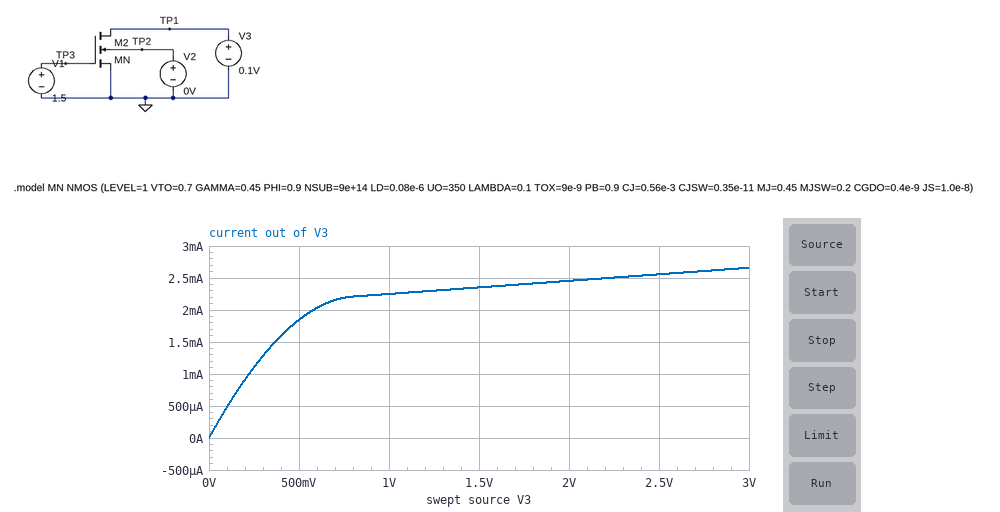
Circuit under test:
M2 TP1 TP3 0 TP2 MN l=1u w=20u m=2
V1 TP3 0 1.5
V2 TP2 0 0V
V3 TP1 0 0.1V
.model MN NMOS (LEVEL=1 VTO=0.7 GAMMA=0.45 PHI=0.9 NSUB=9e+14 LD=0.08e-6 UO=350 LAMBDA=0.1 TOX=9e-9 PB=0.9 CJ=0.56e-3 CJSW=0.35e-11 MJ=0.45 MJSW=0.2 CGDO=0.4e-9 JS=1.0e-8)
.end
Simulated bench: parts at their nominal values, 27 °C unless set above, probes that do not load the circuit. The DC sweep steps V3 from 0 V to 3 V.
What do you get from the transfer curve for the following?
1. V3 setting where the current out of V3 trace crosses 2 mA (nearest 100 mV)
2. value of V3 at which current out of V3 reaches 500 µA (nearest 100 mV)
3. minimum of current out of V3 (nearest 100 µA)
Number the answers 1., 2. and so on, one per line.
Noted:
1. 600 mV
2. 100 mV
3. 0 A
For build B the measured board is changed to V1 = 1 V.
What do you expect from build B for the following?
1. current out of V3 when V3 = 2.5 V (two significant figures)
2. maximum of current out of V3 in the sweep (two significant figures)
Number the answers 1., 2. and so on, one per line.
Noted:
1. 360 µA
2. 370 µA
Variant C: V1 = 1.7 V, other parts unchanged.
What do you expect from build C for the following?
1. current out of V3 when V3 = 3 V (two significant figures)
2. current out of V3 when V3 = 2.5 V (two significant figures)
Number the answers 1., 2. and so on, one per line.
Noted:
1. 4.2 mA
2. 4.0 mA
